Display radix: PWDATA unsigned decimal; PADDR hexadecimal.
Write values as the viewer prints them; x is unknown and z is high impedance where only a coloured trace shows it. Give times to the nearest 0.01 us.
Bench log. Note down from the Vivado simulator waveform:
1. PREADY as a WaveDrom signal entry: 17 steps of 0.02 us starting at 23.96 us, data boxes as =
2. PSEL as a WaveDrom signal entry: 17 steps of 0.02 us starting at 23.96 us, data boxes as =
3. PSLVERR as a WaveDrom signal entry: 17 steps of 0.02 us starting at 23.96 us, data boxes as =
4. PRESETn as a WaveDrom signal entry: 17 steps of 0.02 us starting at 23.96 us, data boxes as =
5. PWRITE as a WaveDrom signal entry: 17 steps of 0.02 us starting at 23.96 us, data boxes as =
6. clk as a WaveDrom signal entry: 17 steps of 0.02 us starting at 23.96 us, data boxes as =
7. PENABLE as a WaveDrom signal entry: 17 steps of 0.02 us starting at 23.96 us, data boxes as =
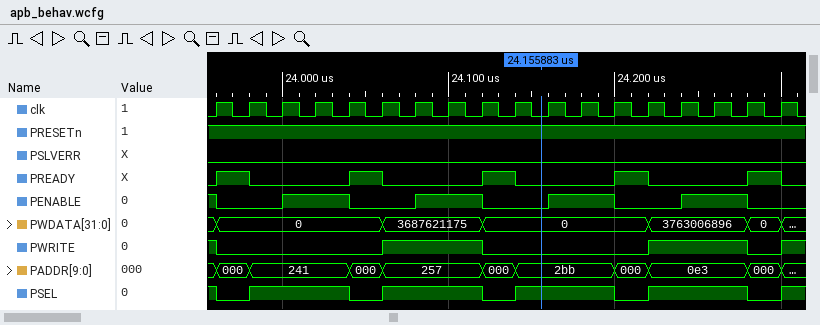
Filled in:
{name: 'PREADY', wave: '10..10..10..10..1'}
{name: 'PSEL', wave: '01..01..01..01..0'}
{name: 'PSLVERR', wave: '0................'}
{name: 'PRESETn', wave: '1................'}
{name: 'PWRITE', wave: '0....1..0....1..0'}
{name: 'clk', wave: 'p................'}
{name: 'PENABLE', wave: '0.1.0.1.0.1.0.1.0'}
